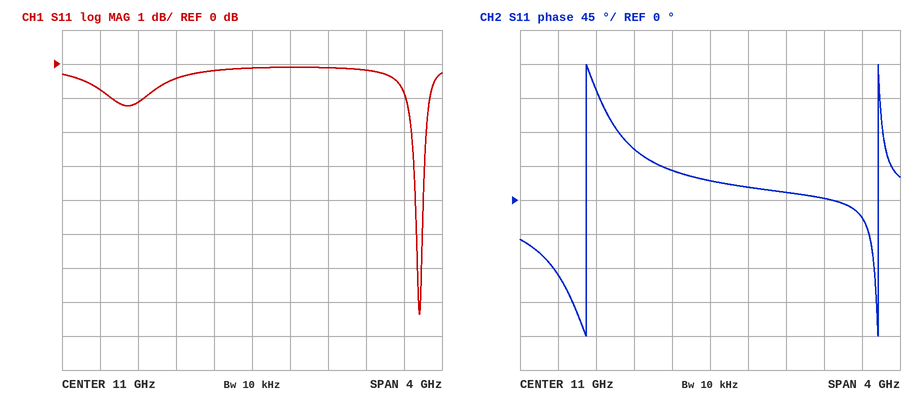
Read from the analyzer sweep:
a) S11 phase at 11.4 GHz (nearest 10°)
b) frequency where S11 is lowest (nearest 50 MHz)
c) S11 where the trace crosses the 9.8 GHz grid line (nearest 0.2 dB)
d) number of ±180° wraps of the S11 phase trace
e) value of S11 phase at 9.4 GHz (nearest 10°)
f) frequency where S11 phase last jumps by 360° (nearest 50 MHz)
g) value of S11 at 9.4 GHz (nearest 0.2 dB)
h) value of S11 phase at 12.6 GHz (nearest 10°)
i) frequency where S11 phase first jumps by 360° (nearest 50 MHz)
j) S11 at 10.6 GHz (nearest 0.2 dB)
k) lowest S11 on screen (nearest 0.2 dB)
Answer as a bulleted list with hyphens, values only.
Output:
- 20°
- 12.75 GHz
- -1.2 dB
- 2
- -100°
- 12.75 GHz
- -0.8 dB
- -20°
- 9.70 GHz
- -0.2 dB
- -7.4 dB
